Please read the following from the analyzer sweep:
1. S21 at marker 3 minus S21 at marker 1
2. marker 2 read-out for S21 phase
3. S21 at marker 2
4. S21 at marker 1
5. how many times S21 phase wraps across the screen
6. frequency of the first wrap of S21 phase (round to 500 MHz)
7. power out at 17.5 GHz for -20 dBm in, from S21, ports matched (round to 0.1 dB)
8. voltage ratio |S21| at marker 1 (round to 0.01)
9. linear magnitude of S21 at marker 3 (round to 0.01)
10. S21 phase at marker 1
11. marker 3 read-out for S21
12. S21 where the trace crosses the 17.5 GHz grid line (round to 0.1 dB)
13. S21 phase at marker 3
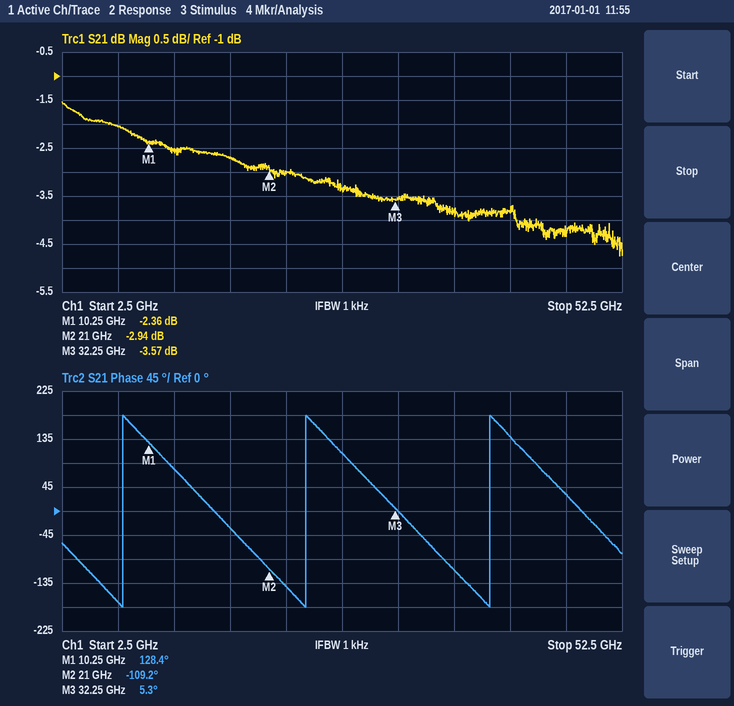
-1.21 dB
-109.2°
-2.94 dB
-2.36 dB
3
8.0 GHz
-22.7 dBm
0.76
0.66
128.4°
-3.57 dB
-2.7 dB
5.3°
